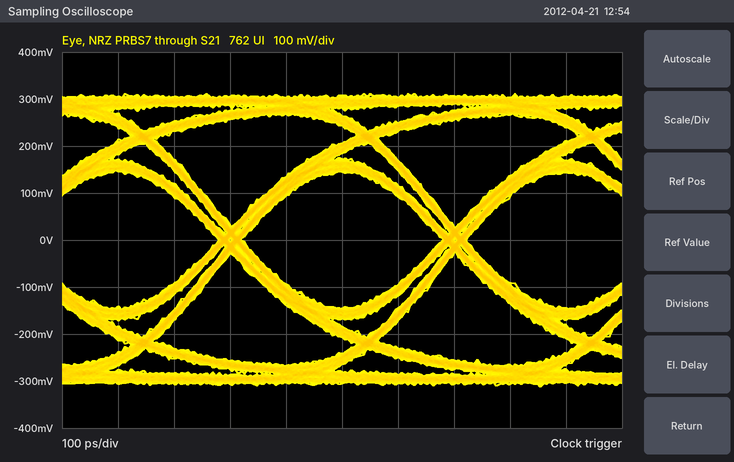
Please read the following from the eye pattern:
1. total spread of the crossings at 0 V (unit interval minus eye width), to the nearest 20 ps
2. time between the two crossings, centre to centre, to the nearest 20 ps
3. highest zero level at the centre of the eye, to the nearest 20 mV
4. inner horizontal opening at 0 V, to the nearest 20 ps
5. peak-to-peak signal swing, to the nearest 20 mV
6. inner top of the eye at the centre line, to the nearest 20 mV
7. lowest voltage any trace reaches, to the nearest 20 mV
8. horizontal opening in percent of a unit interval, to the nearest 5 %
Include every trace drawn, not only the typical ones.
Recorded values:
40 ps
400 ps
-140 mV
360 ps
620 mV
140 mV
-320 mV
90 %
